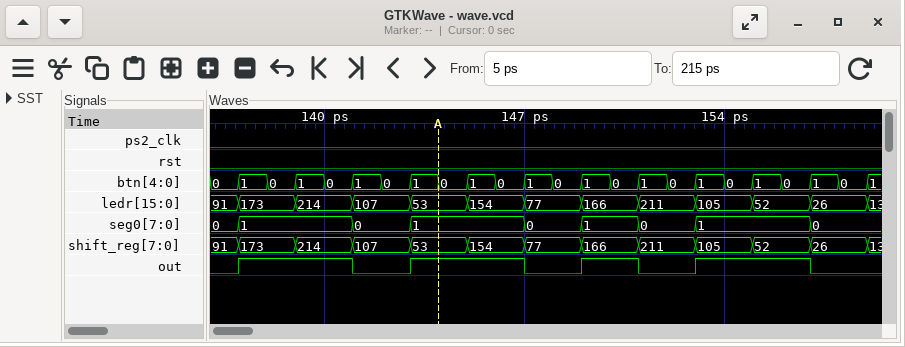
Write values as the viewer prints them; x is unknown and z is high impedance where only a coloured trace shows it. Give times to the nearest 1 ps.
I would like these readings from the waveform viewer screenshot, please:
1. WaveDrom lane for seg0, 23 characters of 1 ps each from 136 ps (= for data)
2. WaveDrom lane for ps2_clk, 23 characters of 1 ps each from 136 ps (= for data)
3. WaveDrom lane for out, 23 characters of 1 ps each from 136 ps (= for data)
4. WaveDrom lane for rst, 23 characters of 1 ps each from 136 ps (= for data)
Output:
{name: 'seg0', wave: '==...=.=...=.=.=.=...=.', data: '0 1 0 1 0 1 0 1 0'}
{name: 'ps2_clk', wave: '0......................'}
{name: 'out', wave: '01...0.1...0.1.0.1...0.'}
{name: 'rst', wave: '0......................'}
